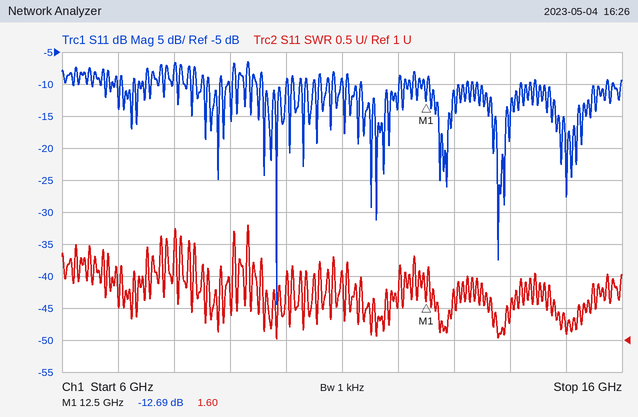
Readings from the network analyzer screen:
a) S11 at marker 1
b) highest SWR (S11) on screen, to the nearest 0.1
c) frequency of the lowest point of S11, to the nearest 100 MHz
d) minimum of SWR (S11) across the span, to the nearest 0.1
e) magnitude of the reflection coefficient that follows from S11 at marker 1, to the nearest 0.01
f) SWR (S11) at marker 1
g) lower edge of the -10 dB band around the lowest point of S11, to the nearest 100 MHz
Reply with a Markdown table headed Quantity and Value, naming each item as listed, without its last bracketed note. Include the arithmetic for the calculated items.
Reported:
| Quantity | Value |
|---|---|
| S11 at marker 1 | -12.69 dB |
| highest SWR (S11) on screen, to the nearest 0.1 | 2.8 |
| frequency of the lowest point of S11, to the nearest 100 MHz | 9.8 GHz |
| minimum of SWR (S11) across the span, to the nearest 0.1 | 1.0 |
| magnitude of the reflection coefficient that follows from S11 at marker 1, to the nearest 0.01 | 10^(-12.69/20) ≈ 0.23 |
| SWR (S11) at marker 1 | 1.60 |
| lower edge of the -10 dB band around the lowest point of S11, to the nearest 100 MHz | 9.6 GHz |
